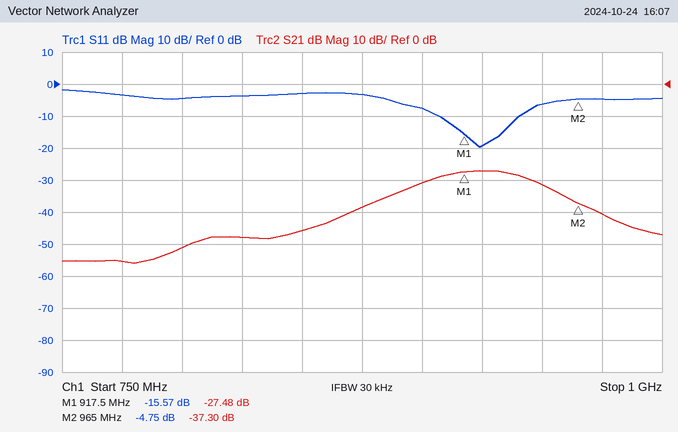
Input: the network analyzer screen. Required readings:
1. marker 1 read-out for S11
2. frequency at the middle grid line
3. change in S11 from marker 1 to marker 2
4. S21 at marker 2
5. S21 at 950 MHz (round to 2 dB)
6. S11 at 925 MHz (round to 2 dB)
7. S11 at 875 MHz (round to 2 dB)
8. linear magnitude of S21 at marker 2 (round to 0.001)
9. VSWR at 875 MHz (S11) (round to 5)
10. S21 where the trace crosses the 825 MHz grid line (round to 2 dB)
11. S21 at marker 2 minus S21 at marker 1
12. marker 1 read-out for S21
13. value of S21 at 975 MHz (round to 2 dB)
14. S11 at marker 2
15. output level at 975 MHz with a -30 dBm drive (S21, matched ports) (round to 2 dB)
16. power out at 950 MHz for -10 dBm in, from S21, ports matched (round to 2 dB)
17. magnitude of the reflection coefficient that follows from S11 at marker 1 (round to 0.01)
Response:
-15.57 dB
875 MHz
10.82 dB
-37.30 dB
-32 dB
-20 dB
-4 dB
0.014
5
-48 dB
-9.82 dB
-27.48 dB
-40 dB
-4.75 dB
-70 dBm
-42 dBm
0.17
